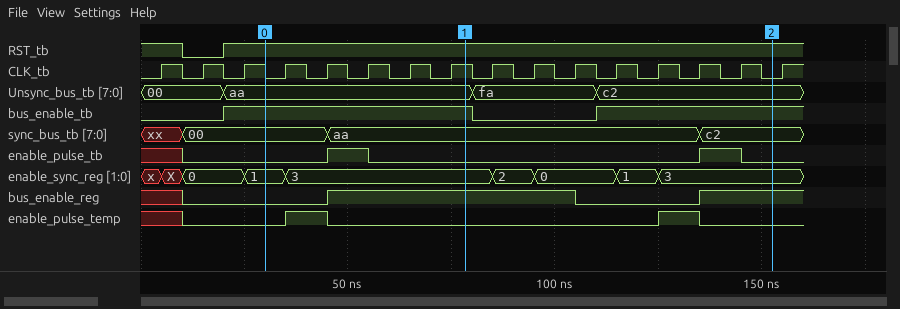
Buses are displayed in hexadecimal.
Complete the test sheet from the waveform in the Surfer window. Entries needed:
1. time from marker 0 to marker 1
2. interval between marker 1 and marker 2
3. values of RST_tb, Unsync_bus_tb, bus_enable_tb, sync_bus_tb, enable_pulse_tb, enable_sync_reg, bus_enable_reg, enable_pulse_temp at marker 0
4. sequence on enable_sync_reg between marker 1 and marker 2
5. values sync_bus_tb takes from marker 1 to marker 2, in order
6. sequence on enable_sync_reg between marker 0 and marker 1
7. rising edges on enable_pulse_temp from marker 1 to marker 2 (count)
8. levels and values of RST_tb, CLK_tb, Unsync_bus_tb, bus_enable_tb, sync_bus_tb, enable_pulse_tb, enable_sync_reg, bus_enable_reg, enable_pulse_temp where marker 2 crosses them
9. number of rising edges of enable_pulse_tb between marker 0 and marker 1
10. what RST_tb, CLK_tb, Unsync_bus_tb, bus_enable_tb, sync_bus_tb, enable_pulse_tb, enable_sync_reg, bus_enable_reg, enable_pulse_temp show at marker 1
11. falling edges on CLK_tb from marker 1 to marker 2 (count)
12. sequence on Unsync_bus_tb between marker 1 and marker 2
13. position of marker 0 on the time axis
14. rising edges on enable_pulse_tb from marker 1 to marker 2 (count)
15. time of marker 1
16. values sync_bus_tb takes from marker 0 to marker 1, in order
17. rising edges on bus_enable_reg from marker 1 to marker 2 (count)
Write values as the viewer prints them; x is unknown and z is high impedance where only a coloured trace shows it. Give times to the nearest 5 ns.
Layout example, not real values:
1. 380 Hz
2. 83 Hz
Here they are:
1. 50 ns
2. 75 ns
3. RST_tb=1, Unsync_bus_tb=aa, bus_enable_tb=1, sync_bus_tb=00, enable_pulse_tb=0, enable_sync_reg=1, bus_enable_reg=0, enable_pulse_temp=0
4. 3, 2, 0, 1, 3
5. aa, c2
6. 1, 3
7. 1
8. RST_tb=1, CLK_tb=0, Unsync_bus_tb=c2, bus_enable_tb=1, sync_bus_tb=c2, enable_pulse_tb=0, enable_sync_reg=3, bus_enable_reg=1, enable_pulse_temp=0
9. 1
10. RST_tb=1, CLK_tb=1, Unsync_bus_tb=aa, bus_enable_tb=1, sync_bus_tb=aa, enable_pulse_tb=0, enable_sync_reg=3, bus_enable_reg=1, enable_pulse_temp=0
11. 8
12. aa, fa, c2
13. 30 ns
14. 1
15. 80 ns
16. 00, aa
17. 1
